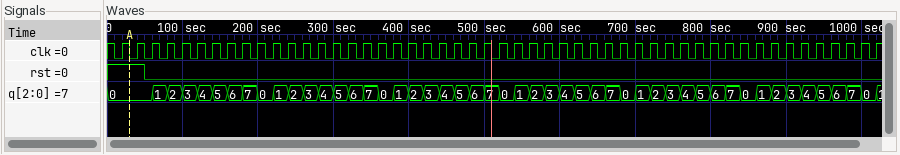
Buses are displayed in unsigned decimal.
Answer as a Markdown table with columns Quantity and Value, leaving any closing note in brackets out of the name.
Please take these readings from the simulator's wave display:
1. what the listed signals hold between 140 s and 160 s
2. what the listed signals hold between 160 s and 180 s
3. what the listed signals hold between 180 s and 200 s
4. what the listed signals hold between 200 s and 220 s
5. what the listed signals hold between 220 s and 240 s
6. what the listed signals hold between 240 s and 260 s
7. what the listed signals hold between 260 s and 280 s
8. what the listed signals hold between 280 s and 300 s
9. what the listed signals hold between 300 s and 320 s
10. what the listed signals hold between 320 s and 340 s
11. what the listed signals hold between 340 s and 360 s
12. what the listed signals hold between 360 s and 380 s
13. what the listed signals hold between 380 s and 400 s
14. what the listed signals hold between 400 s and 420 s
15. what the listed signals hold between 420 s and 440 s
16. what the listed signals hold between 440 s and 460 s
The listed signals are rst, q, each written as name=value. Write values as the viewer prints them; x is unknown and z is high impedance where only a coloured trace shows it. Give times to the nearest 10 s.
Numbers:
| Quantity | Value |
|---|---|
| what the listed signals hold between 140 s and 160 s | rst=0, q=5 |
| what the listed signals hold between 160 s and 180 s | rst=0, q=6 |
| what the listed signals hold between 180 s and 200 s | rst=0, q=7 |
| what the listed signals hold between 200 s and 220 s | rst=0, q=0 |
| what the listed signals hold between 220 s and 240 s | rst=0, q=1 |
| what the listed signals hold between 240 s and 260 s | rst=0, q=2 |
| what the listed signals hold between 260 s and 280 s | rst=0, q=3 |
| what the listed signals hold between 280 s and 300 s | rst=0, q=4 |
| what the listed signals hold between 300 s and 320 s | rst=0, q=5 |
| what the listed signals hold between 320 s and 340 s | rst=0, q=6 |
| what the listed signals hold between 340 s and 360 s | rst=0, q=7 |
| what the listed signals hold between 360 s and 380 s | rst=0, q=0 |
| what the listed signals hold between 380 s and 400 s | rst=0, q=1 |
| what the listed signals hold between 400 s and 420 s | rst=0, q=2 |
| what the listed signals hold between 420 s and 440 s | rst=0, q=3 |
| what the listed signals hold between 440 s and 460 s | rst=0, q=4 |
